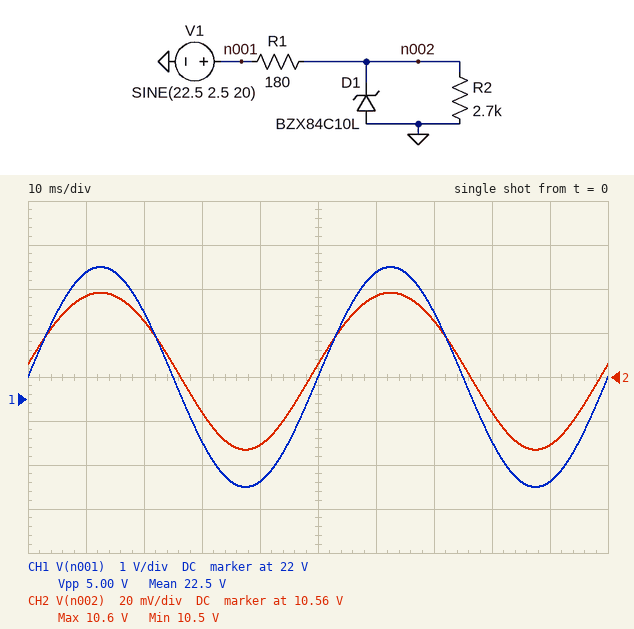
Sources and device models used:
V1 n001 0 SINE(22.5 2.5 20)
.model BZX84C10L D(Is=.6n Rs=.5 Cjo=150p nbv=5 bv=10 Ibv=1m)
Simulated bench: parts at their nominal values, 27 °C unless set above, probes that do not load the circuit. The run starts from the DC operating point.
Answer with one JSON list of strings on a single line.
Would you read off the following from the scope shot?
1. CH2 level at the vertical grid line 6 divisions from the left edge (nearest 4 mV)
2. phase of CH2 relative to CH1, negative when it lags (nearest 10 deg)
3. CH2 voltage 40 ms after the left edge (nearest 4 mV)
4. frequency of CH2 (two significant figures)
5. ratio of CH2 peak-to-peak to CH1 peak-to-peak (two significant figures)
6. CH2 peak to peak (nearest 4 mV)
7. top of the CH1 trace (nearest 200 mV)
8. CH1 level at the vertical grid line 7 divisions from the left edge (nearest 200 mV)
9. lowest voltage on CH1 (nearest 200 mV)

["10.596 V", "0 deg", "10.528 V", "20 Hz", "0.014", "72 mV", "25.0 V", "24.0 V", "20.0 V"]
